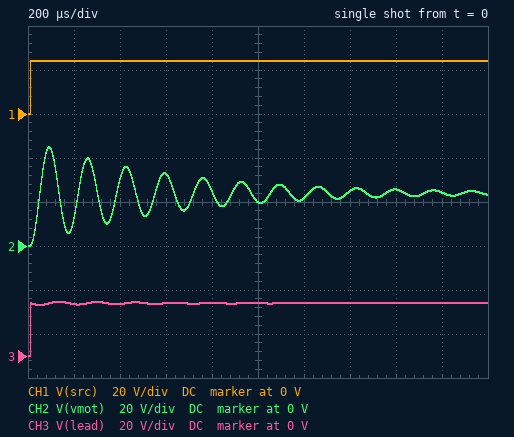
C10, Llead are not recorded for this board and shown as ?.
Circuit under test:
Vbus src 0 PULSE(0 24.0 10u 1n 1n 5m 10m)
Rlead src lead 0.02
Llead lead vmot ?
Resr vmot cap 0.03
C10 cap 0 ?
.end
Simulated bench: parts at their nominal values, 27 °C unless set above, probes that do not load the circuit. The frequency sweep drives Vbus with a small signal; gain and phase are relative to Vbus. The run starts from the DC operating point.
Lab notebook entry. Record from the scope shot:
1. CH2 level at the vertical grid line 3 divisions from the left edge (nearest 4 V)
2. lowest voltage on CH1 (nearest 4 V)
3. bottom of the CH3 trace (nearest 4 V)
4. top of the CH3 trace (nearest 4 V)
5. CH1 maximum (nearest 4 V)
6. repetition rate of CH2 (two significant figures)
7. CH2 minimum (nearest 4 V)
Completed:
32 V
0 V
0 V
24 V
24 V
6.0 kHz
0 V
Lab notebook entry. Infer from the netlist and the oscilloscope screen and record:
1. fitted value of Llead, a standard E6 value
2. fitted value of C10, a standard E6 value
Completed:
15 µH
47 µF
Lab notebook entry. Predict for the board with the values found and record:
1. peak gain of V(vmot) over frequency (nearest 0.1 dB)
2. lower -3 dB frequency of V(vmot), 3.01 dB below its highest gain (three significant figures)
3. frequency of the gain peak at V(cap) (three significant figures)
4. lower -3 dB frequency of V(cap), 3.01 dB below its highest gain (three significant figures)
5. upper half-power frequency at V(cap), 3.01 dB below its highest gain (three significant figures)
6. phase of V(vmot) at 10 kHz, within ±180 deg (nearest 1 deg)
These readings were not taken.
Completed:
21.1 dB
5.71 kHz
5.98 kHz
5.71 kHz
6.24 kHz
-170 deg
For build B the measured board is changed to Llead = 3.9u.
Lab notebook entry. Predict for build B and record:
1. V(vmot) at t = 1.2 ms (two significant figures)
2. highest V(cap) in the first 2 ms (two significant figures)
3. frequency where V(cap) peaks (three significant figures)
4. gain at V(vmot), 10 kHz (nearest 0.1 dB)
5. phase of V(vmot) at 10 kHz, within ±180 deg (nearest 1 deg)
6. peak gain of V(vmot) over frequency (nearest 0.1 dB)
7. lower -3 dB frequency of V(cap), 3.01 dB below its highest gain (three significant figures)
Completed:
24 V
42 V
11.7 kHz
10.1 dB
-23 deg
15.3 dB
10.6 kHz
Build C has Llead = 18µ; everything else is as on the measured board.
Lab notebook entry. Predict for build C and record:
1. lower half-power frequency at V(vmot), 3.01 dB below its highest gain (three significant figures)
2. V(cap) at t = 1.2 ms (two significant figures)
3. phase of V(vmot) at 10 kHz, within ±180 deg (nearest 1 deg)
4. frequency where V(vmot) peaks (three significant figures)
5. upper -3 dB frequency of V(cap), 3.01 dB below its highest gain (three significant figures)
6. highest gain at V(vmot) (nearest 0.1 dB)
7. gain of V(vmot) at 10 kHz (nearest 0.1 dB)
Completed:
5.24 kHz
29 V
-171 deg
5.46 kHz
5.68 kHz
21.9 dB
-7.4 dB
